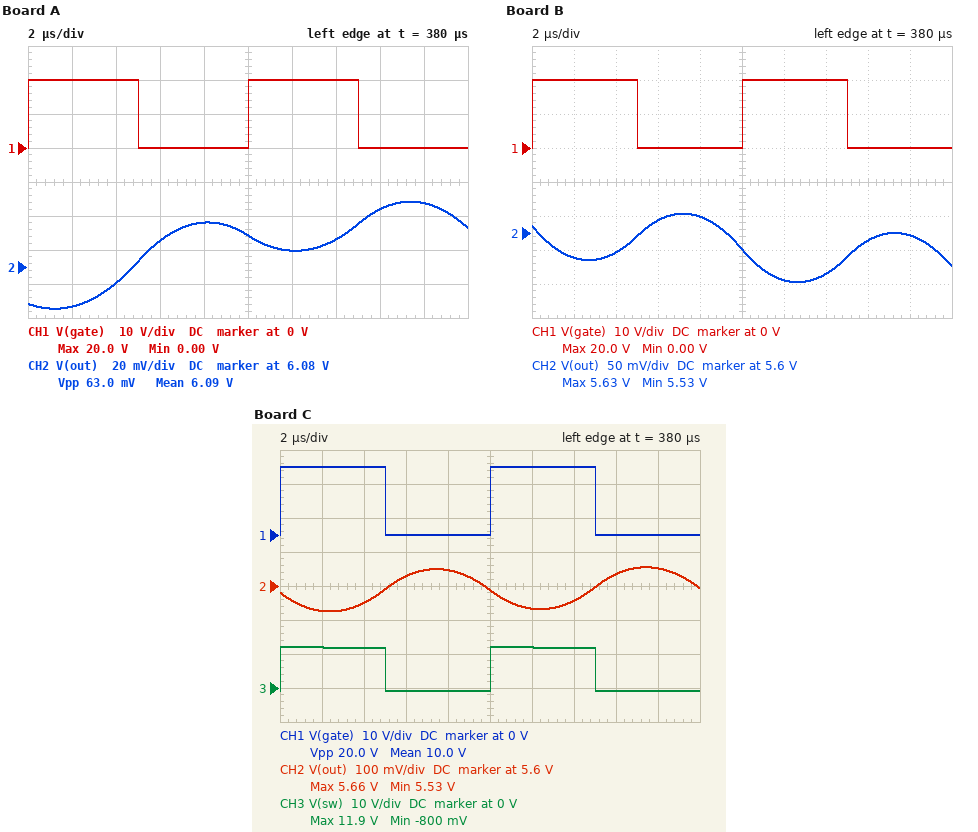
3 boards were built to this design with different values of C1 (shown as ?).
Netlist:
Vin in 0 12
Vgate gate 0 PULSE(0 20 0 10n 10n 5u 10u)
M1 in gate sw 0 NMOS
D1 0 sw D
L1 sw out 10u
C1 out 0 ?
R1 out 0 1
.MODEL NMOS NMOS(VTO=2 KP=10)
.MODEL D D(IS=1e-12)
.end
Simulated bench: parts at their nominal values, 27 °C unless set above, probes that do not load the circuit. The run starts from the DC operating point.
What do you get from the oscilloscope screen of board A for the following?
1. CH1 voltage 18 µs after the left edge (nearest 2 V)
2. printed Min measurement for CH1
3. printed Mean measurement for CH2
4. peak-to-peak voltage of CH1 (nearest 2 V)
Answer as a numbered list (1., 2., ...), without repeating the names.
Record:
1. 0 V
2. 0.00 V
3. 6.09 V
4. 20 V
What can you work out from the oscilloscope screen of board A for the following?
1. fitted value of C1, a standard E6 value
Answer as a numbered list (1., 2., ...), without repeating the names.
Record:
1. 150 µF
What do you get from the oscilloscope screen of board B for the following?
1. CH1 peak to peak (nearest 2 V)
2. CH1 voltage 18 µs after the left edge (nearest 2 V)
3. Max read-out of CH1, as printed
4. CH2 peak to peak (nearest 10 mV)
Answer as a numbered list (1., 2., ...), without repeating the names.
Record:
1. 20 V
2. 0 V
3. 20.0 V
4. 100 mV
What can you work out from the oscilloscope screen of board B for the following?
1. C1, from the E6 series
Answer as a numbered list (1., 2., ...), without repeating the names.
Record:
1. 47 µF
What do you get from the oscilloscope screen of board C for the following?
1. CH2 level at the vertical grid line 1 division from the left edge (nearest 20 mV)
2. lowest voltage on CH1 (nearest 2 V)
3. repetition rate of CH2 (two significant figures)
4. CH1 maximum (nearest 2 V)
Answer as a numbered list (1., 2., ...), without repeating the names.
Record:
1. 5.52 V
2. 0 V
3. 100 kHz
4. 20 V
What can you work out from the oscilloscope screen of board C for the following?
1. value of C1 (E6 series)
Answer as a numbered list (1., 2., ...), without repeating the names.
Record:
1. 33 µF
